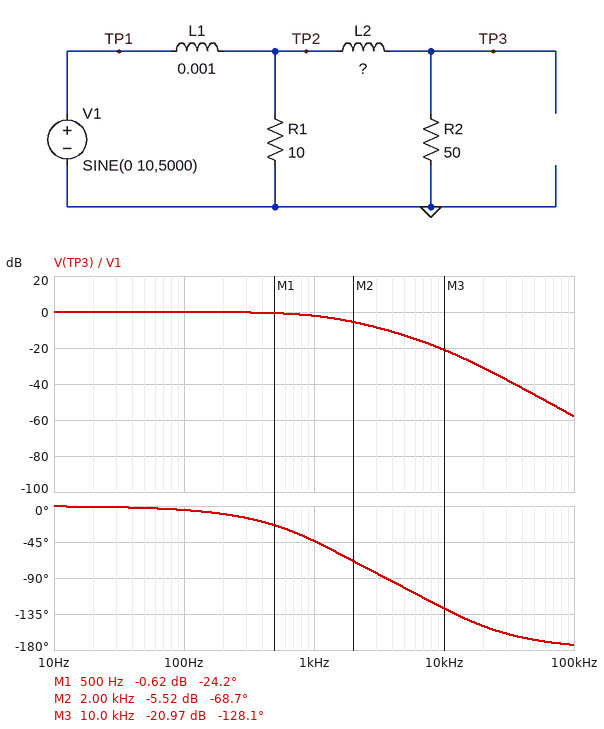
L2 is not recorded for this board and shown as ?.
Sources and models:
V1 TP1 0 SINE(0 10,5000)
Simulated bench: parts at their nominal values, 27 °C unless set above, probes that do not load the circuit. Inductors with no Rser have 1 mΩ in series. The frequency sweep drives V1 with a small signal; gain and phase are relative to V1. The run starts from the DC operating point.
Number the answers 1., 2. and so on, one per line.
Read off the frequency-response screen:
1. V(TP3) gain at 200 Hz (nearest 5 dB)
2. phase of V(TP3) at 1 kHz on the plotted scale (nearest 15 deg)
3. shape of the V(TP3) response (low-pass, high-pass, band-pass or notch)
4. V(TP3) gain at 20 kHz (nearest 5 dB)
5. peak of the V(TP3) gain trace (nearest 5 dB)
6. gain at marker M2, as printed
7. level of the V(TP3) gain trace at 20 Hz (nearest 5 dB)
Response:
1. 0 dB
2. -45 deg
3. low-pass
4. -30 dB
5. 0 dB
6. -5.52 dB
7. 0 dB
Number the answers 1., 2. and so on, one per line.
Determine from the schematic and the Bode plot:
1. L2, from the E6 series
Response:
1. 1 mH
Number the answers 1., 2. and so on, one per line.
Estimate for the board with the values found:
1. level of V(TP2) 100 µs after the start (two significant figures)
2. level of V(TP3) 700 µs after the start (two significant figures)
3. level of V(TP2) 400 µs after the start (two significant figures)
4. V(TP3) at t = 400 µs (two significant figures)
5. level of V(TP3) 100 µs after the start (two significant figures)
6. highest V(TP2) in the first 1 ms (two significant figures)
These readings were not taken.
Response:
1. 3.5 V
2. 2.2 V
3. -2.4 V
4. -2.1 V
5. 3.4 V
6. 3.8 V
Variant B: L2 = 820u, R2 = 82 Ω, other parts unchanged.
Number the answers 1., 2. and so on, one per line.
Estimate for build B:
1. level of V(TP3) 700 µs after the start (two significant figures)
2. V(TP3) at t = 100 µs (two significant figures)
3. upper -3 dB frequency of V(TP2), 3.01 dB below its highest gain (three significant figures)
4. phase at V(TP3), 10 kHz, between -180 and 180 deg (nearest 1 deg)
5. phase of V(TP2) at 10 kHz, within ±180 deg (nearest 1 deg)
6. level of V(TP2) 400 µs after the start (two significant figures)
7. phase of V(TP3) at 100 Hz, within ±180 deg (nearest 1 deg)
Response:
1. 2.6 V
2. 3.8 V
3. 1.41 kHz
4. -111 deg
5. -79 deg
6. -2.5 V
7. -4 deg
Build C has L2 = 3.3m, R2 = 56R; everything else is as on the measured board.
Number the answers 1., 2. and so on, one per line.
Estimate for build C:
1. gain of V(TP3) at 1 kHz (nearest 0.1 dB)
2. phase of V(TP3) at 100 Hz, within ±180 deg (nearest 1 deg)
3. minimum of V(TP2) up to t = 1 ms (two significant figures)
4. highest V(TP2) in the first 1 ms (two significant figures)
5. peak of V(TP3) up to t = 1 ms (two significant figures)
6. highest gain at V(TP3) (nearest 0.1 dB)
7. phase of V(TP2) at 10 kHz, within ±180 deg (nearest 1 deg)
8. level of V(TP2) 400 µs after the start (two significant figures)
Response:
1. -2.6 dB
2. -6 deg
3. -2.9 V
4. 4.0 V
5. 2.6 V
6. 0 dB
7. -79 deg
8. -2.6 V
